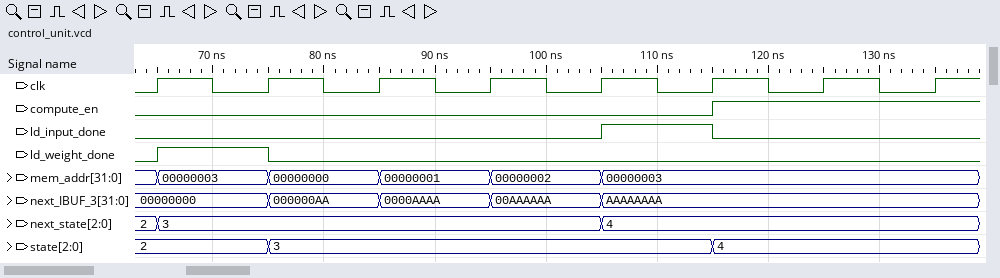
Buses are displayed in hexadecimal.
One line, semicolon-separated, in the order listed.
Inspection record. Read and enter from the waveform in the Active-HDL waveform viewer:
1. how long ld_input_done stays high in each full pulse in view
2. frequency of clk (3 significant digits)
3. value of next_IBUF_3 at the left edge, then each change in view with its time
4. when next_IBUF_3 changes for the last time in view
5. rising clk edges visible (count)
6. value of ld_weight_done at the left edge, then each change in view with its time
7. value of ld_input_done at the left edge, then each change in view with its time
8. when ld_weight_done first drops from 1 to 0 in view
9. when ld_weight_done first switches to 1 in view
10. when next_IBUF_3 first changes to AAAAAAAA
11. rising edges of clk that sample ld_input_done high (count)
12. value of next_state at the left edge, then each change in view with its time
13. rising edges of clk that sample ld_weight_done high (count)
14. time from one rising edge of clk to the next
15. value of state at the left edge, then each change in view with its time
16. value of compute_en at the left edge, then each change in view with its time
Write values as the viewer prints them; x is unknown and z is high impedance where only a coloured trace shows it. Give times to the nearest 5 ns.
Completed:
10 ns; 100 MHz; 00000000, 000000AA at 75 ns, 0000AAAA at 85 ns, 00AAAAAA at 95 ns, AAAAAAAA at 105 ns; 105 ns; 8; 0, 1 at 65 ns, 0 at 75 ns; 0, 1 at 105 ns, 0 at 115 ns; 75 ns; 65 ns; 105 ns; 1; 2, 3 at 65 ns, 4 at 105 ns; 1; 10 ns; 2, 3 at 75 ns, 4 at 115 ns; 0, 1 at 115 ns
